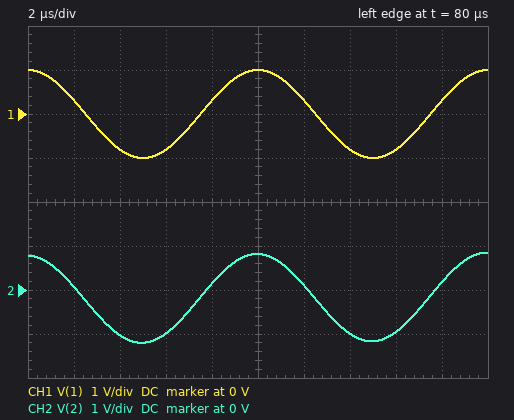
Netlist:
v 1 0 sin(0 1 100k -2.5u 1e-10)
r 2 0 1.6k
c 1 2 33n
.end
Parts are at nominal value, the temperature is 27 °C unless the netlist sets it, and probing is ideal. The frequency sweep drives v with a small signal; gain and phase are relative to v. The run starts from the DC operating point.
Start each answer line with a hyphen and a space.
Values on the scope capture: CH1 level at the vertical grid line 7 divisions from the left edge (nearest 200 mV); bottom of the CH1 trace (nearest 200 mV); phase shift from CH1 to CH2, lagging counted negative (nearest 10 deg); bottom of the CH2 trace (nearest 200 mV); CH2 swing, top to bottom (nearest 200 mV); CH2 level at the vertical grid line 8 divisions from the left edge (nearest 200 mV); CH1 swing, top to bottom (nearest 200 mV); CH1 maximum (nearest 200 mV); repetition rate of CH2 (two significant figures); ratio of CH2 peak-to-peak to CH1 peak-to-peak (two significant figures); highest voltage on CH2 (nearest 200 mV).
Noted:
- -800 mV
- -1.0 V
- 0 deg
- -1.2 V
- 2.0 V
- -1.0 V
- 2.0 V
- 1.0 V
- 100 kHz
- 1.0
- 800 mV
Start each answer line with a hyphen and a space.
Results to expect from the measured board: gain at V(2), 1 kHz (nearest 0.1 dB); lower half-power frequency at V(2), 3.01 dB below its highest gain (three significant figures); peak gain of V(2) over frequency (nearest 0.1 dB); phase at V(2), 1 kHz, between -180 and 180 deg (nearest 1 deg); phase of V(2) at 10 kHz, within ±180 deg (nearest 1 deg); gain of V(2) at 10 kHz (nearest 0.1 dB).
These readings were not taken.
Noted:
- -10.0 dB
- 3.01 kHz
- 0 dB
- 72 deg
- 17 deg
- -0.4 dB
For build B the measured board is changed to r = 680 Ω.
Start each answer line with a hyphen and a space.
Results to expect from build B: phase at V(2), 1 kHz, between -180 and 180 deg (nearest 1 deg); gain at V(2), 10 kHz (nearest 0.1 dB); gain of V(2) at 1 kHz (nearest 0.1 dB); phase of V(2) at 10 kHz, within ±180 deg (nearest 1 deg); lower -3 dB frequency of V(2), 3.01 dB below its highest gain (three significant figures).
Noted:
- 82 deg
- -1.8 dB
- -17.1 dB
- 35 deg
- 7.09 kHz
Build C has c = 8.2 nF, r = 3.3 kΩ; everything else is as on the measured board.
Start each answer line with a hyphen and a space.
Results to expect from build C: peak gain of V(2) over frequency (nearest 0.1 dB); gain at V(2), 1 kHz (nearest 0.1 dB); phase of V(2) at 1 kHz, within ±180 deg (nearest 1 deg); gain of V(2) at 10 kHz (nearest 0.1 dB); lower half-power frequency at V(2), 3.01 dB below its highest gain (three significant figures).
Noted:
- 0 dB
- -15.5 dB
- 80 deg
- -1.3 dB
- 5.88 kHz
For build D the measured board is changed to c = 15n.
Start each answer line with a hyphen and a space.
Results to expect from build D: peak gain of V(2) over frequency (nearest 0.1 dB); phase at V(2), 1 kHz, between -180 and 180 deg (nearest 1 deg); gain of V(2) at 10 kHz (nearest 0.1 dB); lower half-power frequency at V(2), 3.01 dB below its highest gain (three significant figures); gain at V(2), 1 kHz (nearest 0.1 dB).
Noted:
- 0 dB
- 81 deg
- -1.6 dB
- 6.63 kHz
- -16.5 dB
